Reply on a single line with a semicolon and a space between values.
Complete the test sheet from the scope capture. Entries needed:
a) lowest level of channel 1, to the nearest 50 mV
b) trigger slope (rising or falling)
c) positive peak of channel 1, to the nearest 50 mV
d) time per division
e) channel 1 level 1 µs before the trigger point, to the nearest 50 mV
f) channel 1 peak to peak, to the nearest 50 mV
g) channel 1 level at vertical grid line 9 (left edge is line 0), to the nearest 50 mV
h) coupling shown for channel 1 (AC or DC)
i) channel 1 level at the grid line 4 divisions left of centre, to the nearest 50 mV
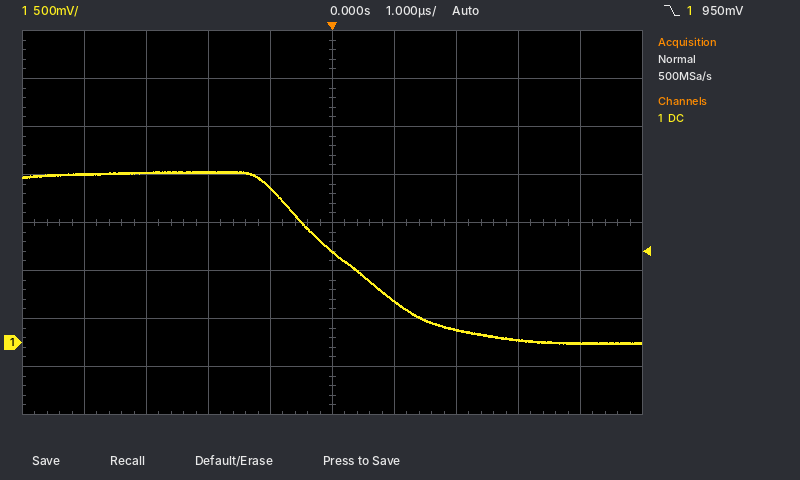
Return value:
0 mV; falling; 1.80 V; 1 µs; 1.60 V; 1.80 V; 0 mV; DC; 1.75 V
